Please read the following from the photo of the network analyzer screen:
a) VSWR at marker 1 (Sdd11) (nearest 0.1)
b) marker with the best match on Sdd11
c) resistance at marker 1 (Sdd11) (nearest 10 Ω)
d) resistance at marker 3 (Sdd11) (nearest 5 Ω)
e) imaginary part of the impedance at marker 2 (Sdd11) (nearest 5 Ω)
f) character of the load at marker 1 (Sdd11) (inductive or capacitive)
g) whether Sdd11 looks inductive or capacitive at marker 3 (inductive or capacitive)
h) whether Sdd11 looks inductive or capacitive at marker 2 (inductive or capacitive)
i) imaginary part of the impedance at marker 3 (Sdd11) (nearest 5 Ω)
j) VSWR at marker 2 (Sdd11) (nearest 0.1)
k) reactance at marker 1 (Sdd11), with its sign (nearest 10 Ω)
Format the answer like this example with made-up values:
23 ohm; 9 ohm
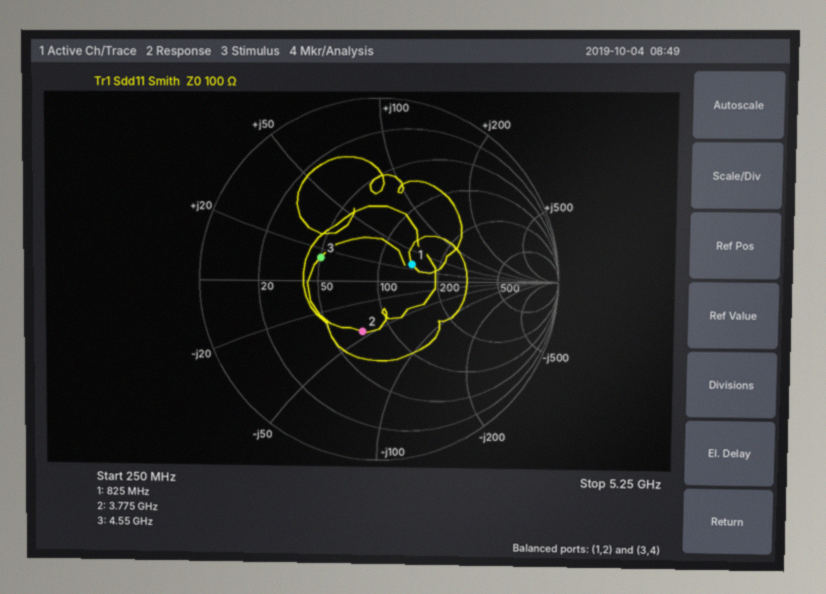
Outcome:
1.5; marker 1; 140 Ω; 50 Ω; -45 Ω; inductive; inductive; capacitive; +15 Ω; 1.8; +30 Ω
